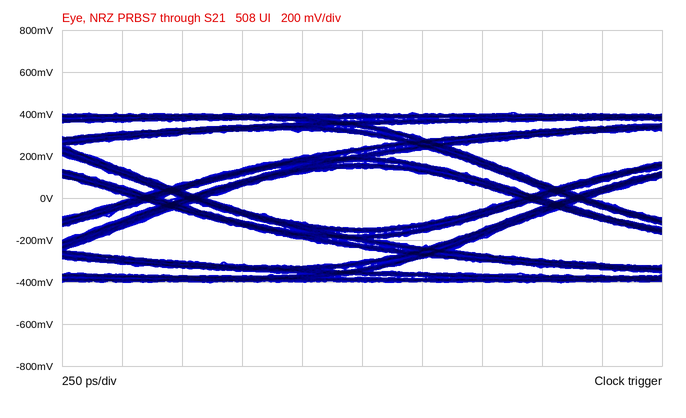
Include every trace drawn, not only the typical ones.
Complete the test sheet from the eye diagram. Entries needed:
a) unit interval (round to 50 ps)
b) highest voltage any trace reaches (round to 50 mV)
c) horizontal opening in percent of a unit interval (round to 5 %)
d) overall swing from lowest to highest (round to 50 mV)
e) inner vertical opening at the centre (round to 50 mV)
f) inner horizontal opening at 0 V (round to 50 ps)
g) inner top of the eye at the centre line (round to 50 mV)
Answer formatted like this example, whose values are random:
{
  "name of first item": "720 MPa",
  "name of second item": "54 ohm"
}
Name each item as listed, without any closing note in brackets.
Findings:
{
  "unit interval": "1.60 ns",
  "highest voltage any trace reaches": "400 mV",
  "horizontal opening in percent of a unit interval": "80 %",
  "overall swing from lowest to highest": "800 mV",
  "inner vertical opening at the centre": "300 mV",
  "inner horizontal opening at 0 V": "1.30 ns",
  "inner top of the eye at the centre line": "150 mV"
}
